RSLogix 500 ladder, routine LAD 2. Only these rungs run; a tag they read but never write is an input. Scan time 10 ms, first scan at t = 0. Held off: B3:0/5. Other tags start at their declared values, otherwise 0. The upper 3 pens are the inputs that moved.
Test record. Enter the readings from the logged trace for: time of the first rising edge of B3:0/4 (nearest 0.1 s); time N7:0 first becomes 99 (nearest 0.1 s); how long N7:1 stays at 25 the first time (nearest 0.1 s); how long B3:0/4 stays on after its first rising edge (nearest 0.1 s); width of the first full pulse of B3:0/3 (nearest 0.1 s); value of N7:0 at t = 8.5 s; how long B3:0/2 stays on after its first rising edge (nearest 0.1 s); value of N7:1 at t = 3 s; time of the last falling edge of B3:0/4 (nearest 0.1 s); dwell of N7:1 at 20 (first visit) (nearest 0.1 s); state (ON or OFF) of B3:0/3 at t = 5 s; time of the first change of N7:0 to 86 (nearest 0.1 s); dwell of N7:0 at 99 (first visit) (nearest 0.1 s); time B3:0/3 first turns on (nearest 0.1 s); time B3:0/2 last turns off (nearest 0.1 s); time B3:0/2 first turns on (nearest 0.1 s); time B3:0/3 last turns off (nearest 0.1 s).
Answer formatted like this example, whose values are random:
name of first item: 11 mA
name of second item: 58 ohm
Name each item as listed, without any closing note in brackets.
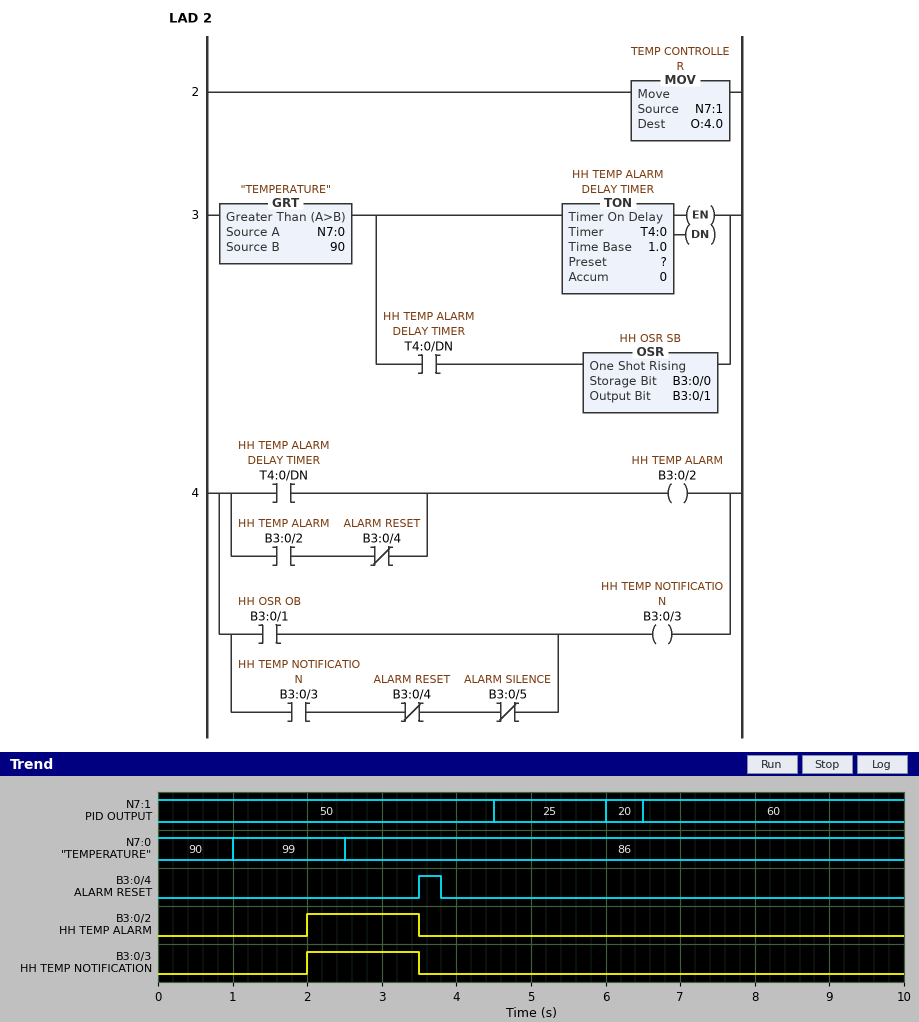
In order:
time of the first rising edge of B3:0/4: 3.5 s
time N7:0 first becomes 99: 1.0 s
how long N7:1 stays at 25 the first time: 1.5 s
how long B3:0/4 stays on after its first rising edge: 0.3 s
width of the first full pulse of B3:0/3: 1.5 s
value of N7:0 at t = 8.5 s: 86
how long B3:0/2 stays on after its first rising edge: 1.5 s
value of N7:1 at t = 3 s: 50
time of the last falling edge of B3:0/4: 3.8 s
dwell of N7:1 at 20 (first visit): 0.5 s
state (ON or OFF) of B3:0/3 at t = 5 s: OFF
time of the first change of N7:0 to 86: 2.5 s
dwell of N7:0 at 99 (first visit): 1.5 s
time B3:0/3 first turns on: 2.0 s
time B3:0/2 last turns off: 3.5 s
time B3:0/2 first turns on: 2.0 s
time B3:0/3 last turns off: 3.5 s
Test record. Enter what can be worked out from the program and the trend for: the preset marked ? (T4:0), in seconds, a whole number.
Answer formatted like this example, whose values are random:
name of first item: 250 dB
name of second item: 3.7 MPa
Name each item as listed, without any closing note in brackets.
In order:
the preset marked ? (T4:0), in seconds, a whole number: 1 s
